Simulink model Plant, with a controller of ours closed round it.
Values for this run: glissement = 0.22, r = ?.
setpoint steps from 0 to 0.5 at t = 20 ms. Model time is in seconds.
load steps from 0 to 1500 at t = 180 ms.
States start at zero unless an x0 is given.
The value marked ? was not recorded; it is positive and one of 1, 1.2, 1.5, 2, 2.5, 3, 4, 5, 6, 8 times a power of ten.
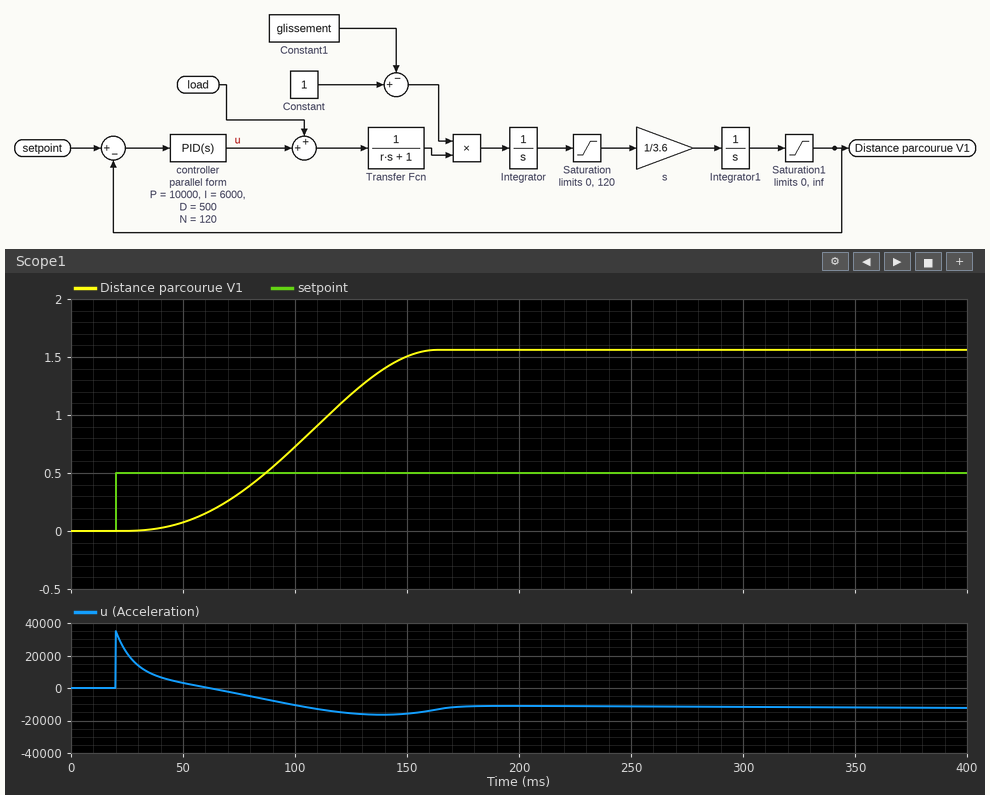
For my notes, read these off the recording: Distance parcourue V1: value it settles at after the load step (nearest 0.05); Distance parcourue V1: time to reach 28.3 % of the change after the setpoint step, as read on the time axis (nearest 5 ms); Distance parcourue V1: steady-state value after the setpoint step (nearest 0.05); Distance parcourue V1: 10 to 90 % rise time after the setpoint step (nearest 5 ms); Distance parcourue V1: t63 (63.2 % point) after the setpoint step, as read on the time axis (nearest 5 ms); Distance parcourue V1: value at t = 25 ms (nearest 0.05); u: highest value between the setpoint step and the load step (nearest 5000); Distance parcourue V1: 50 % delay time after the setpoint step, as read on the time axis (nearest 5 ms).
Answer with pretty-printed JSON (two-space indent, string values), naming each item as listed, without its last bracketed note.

{
  "Distance parcourue V1: value it settles at after the load step": "1.55",
  "Distance parcourue V1: time to reach 28.3 % of the change after the setpoint step, as read on the time axis": "85 ms",
  "Distance parcourue V1: steady-state value after the setpoint step": "1.55",
  "Distance parcourue V1: 10 to 90 % rise time after the setpoint step": "80 ms",
  "Distance parcourue V1: t63 (63.2 % point) after the setpoint step, as read on the time axis": "115 ms",
  "Distance parcourue V1: value at t = 25 ms": "0.00",
  "u: highest value between the setpoint step and the load step": "35000",
  "Distance parcourue V1: 50 % delay time after the setpoint step, as read on the time axis": "105 ms"
}
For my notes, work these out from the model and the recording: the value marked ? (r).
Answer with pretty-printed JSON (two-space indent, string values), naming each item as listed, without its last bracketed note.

{
  "the value marked ?": "0.25"
}
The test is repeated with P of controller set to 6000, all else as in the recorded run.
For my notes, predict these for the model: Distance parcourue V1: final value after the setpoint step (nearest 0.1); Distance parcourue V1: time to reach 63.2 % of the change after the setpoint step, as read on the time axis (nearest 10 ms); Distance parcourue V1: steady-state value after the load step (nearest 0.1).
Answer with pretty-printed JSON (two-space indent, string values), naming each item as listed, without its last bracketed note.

{
  "Distance parcourue V1: final value after the setpoint step": "1.4",
  "Distance parcourue V1: time to reach 63.2 % of the change after the setpoint step, as read on the time axis": "120 ms",
  "Distance parcourue V1: steady-state value after the load step": "1.4"
}
